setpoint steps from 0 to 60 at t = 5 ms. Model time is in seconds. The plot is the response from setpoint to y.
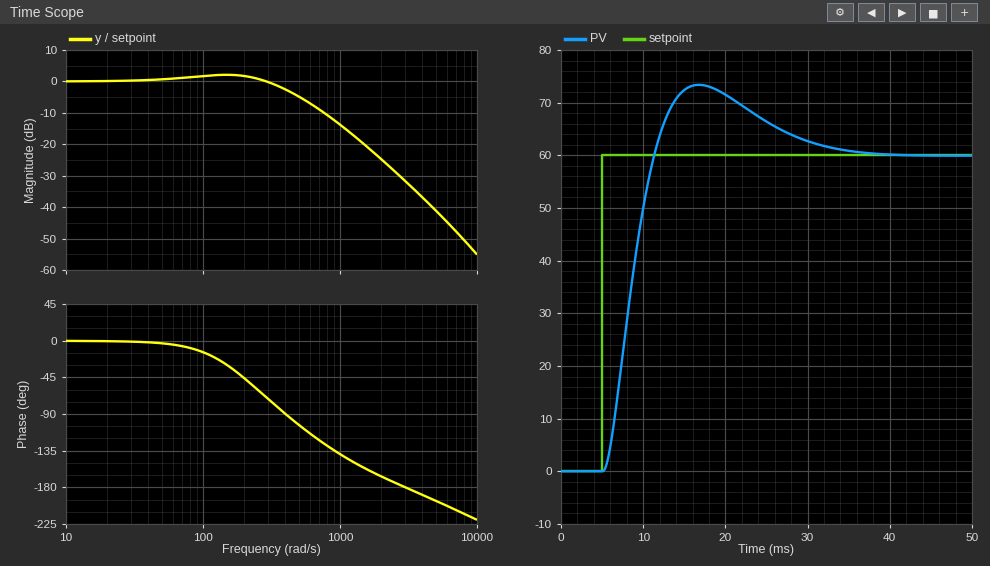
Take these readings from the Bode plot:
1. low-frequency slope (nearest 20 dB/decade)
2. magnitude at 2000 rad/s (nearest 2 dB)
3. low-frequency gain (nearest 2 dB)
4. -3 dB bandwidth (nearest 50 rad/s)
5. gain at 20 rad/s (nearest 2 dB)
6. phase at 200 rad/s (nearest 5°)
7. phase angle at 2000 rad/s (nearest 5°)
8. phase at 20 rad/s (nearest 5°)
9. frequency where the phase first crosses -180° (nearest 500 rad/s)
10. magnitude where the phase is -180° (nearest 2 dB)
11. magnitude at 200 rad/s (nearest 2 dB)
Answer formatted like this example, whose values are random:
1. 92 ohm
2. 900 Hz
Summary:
1. 0 dB/decade
2. -24 dB
3. 0 dB
4. 400 rad/s
5. 0 dB
6. -45°
7. -165°
8. 0°
9. 3000 rad/s
10. -32 dB
11. 2 dB
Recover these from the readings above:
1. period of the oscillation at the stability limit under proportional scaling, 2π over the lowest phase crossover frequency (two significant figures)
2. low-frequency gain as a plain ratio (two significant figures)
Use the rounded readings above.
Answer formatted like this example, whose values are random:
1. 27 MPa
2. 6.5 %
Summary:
1. 0.0021 s
2. 1.0
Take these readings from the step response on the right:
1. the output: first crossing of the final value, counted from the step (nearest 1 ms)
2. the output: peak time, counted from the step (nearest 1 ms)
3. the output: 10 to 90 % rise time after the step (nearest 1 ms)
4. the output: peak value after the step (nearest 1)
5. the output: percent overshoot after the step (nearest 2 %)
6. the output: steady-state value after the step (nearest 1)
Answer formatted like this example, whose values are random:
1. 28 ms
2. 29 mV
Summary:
1. 6 ms
2. 12 ms
3. 4 ms
4. 73
5. 22 %
6. 60
